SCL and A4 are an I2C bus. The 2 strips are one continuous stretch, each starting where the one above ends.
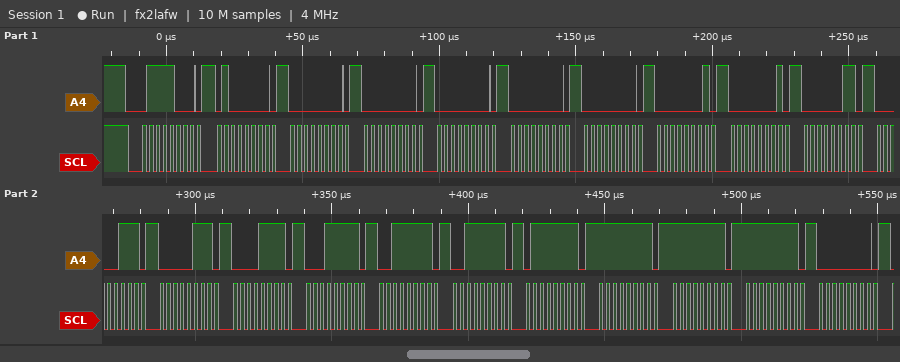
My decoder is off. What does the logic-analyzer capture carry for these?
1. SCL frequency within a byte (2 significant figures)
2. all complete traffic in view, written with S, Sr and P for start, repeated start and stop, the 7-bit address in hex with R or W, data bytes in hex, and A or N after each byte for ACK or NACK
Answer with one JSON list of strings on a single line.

["400 kHz", "S 3CW A 40 A 00 A 00 A 00 A 00 A 00 A 01 A 01 A 03 A 07 A 07 A 0F A 1F A 3F A 3F A 7F A FF A FF A FF A 00 A"]
